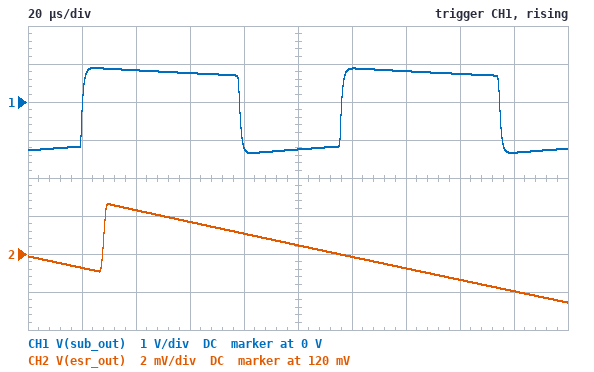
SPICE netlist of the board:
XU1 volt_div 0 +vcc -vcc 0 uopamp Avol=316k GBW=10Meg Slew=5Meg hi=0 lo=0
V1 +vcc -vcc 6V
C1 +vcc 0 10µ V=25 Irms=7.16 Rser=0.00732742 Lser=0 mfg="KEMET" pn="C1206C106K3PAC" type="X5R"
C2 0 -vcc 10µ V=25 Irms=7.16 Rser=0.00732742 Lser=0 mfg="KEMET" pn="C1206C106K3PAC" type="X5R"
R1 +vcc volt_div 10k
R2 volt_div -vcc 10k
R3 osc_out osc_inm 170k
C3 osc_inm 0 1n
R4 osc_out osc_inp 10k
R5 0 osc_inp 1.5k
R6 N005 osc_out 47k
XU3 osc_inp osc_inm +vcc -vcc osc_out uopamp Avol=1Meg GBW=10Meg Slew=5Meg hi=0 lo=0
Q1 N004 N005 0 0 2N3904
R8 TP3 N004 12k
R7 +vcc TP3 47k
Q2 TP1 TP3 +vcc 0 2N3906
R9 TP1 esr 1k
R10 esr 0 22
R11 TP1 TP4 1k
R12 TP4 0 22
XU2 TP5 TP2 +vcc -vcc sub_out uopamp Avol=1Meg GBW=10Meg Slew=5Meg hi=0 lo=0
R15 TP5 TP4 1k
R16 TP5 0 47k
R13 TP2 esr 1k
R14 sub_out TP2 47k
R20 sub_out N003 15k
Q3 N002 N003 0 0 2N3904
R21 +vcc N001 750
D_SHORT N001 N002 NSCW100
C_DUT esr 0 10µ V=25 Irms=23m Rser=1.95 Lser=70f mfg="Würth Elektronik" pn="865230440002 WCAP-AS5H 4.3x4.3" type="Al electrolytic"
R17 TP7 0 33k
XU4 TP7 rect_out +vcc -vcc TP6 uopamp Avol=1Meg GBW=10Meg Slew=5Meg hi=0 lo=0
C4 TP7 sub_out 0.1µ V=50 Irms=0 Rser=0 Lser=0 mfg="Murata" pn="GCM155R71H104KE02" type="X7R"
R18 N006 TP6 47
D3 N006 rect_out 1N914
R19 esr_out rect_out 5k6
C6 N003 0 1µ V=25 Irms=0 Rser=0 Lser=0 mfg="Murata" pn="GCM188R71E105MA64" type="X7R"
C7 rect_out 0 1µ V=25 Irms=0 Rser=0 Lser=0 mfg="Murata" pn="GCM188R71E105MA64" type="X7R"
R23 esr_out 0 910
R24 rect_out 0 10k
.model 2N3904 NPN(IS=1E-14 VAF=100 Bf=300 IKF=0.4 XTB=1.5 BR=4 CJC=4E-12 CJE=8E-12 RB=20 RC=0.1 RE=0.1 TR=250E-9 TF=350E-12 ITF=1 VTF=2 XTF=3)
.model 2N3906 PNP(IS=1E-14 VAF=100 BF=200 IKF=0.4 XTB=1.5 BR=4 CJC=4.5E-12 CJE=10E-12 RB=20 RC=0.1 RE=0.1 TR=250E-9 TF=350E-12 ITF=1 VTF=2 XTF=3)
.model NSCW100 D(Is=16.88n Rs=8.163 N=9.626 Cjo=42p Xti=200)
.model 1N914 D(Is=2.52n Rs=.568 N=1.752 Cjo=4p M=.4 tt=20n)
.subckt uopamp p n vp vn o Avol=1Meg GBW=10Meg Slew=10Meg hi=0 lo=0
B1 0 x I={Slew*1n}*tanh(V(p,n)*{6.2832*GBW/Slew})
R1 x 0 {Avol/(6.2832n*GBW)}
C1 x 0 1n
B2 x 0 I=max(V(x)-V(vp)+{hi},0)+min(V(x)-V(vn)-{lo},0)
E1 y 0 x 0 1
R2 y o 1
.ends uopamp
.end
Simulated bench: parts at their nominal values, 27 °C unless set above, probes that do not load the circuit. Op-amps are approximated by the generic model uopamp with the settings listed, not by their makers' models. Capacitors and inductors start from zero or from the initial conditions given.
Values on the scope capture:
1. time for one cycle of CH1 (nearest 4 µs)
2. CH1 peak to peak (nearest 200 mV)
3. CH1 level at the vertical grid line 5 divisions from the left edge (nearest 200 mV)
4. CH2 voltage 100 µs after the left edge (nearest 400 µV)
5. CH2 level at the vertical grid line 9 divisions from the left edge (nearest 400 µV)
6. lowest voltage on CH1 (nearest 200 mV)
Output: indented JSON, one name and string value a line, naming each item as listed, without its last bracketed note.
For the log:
{
  "time for one cycle of CH1": "96 µs",
  "CH1 peak to peak": "2.2 V",
  "CH1 level at the vertical grid line 5 divisions from the left edge": "-1.2 V",
  "CH2 voltage 100 µs after the left edge": "120.4 mV",
  "CH2 level at the vertical grid line 9 divisions from the left edge": "118.0 mV",
  "lowest voltage on CH1": "-1.4 V"
}
